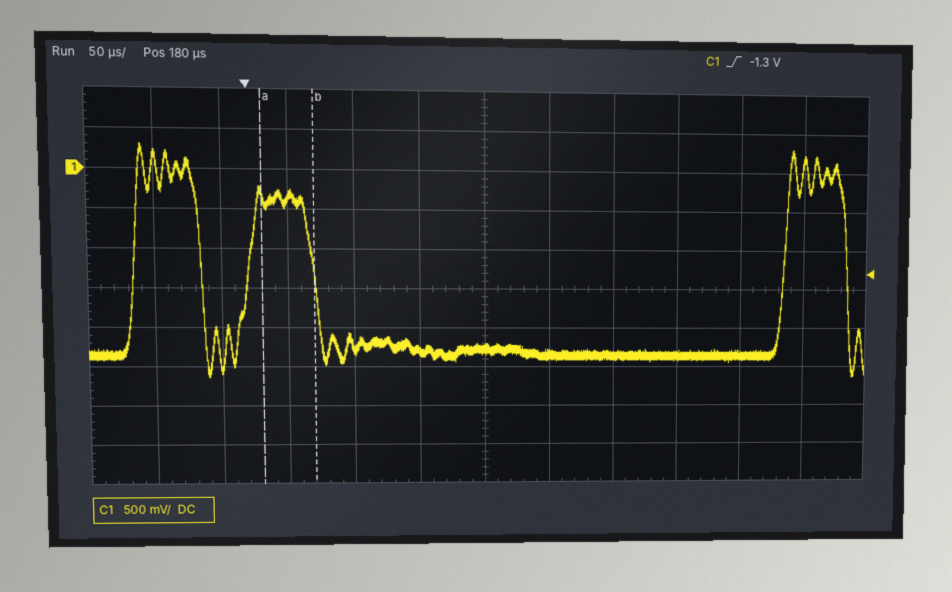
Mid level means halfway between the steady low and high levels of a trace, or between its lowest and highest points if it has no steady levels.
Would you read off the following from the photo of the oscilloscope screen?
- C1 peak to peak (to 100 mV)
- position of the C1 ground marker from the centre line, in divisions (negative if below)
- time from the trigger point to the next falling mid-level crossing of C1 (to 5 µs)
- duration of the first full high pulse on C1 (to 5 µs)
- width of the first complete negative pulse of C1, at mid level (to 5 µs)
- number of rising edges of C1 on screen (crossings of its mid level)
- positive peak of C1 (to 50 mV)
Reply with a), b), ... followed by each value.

a) 2.90 V
b) +3.0 div
c) 50 µs
d) 50 µs
e) 35 µs
f) 3
g) 300 mV
